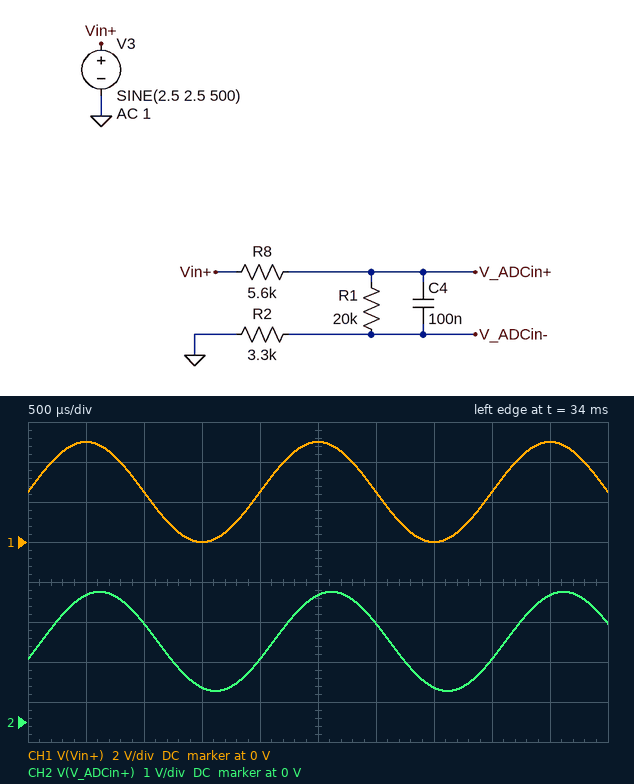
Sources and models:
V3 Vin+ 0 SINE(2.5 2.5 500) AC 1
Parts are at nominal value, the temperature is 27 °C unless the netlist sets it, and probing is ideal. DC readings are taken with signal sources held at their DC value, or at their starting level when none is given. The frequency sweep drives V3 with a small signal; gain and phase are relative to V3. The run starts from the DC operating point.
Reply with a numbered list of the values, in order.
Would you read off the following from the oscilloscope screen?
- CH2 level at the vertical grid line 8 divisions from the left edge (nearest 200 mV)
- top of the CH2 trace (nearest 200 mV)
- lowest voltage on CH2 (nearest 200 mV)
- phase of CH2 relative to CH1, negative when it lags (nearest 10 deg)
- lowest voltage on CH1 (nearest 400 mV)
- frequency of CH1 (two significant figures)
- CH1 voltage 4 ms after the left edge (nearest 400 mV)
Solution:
1. 1.6 V
2. 3.2 V
3. 800 mV
4. -20 deg
5. 0 V
6. 500 Hz
7. 2.4 V
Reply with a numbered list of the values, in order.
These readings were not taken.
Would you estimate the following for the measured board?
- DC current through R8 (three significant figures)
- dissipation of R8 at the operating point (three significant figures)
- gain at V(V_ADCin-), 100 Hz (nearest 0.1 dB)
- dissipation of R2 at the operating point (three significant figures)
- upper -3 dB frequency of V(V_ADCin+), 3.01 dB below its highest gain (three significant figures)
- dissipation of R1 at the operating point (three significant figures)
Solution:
1. 86.5 µA
2. 41.9 µW
3. -15.3 dB
4. 24.7 µW
5. 340 Hz
6. 150 µW
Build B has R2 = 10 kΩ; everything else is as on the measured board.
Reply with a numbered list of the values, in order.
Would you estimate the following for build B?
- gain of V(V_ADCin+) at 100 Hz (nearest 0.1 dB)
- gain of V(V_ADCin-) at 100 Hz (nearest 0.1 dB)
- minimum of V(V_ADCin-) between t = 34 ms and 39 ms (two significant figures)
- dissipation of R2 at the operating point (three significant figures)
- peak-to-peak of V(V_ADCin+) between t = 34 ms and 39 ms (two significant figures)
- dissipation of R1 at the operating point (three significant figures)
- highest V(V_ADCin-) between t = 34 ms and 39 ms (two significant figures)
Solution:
1. -1.9 dB
2. -8.1 dB
3. -820 mV
4. 49.3 µW
5. 3.3 V
6. 98.6 µW
7. 2.2 V
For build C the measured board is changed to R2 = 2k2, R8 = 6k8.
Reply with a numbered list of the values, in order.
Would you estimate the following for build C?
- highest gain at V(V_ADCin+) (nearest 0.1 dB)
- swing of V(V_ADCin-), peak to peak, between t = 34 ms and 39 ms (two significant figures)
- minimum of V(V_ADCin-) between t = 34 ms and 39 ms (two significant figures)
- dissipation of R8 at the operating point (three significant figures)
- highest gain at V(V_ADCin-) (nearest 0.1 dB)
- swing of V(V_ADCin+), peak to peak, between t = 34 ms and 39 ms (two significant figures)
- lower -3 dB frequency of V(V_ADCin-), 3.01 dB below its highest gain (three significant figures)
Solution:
1. -2.3 dB
2. 1.1 V
3. -360 mV
4. 50.5 µW
5. -12.2 dB
6. 2.1 V
7. 230 Hz
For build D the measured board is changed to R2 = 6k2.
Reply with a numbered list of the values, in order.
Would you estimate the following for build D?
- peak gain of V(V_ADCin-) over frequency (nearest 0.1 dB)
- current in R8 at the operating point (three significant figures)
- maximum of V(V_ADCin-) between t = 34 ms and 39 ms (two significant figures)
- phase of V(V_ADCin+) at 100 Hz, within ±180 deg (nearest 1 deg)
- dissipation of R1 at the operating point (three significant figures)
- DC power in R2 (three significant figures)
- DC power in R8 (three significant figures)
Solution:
1. -5.6 dB
2. 78.6 µA
3. 1.7 V
4. -8 deg
5. 124 µW
6. 38.3 µW
7. 34.6 µW
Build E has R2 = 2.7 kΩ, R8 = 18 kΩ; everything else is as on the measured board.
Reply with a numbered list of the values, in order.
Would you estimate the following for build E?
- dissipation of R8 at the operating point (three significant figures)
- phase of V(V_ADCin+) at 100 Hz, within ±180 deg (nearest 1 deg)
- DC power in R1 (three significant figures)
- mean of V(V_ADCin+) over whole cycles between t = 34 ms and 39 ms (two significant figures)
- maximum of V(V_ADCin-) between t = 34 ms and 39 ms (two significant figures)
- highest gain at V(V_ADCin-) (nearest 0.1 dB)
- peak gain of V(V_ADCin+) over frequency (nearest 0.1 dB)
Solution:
1. 67.9 µW
2. -24 deg
3. 75.5 µW
4. 1.4 V
5. 480 mV
6. -17.7 dB
7. -5.1 dB
